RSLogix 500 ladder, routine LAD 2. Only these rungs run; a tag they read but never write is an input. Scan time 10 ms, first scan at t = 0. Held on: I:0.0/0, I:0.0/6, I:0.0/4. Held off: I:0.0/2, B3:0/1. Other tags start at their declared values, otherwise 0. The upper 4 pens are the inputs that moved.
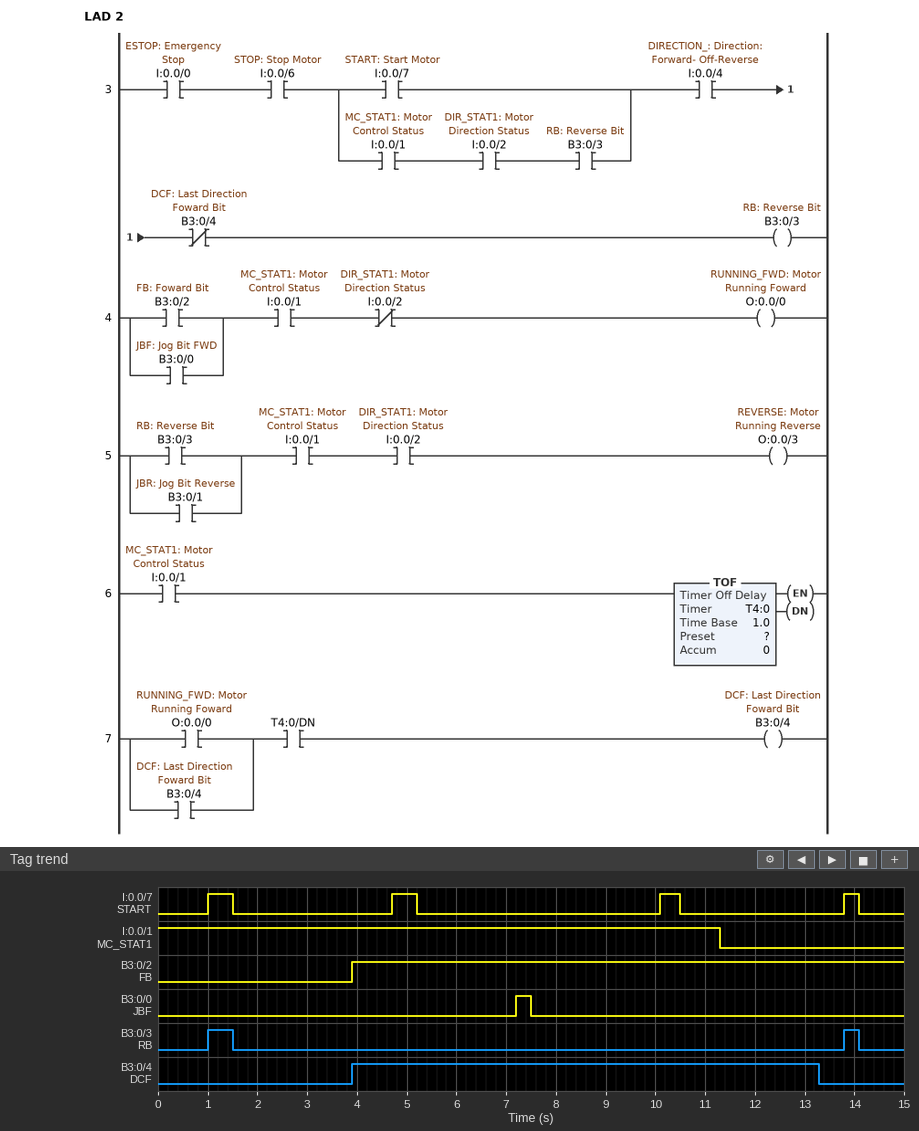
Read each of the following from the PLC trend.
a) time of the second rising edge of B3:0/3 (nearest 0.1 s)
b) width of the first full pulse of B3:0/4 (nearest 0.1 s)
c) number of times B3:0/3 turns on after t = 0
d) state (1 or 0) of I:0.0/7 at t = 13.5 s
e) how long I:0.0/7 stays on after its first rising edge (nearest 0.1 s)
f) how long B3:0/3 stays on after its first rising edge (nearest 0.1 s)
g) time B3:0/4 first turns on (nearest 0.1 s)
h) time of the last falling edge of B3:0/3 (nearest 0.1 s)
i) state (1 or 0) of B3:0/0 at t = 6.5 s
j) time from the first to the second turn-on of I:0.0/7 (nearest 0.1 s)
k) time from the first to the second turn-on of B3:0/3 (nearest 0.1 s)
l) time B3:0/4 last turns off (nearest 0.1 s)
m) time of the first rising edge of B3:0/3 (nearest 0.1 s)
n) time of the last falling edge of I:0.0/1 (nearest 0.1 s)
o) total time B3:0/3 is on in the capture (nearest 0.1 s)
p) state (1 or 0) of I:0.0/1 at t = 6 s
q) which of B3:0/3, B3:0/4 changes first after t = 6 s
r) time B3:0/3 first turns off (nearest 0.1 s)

13.8 s
9.4 s
2
0
0.5 s
0.5 s
3.9 s
14.1 s
0
3.7 s
12.8 s
13.3 s
1.0 s
11.3 s
0.8 s
1
B3:0/4
1.5 s
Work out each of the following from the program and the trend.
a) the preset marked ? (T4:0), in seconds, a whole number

2 s
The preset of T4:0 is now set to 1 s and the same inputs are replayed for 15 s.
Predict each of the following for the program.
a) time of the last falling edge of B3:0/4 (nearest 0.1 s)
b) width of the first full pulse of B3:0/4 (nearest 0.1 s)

12.3 s
8.4 s
